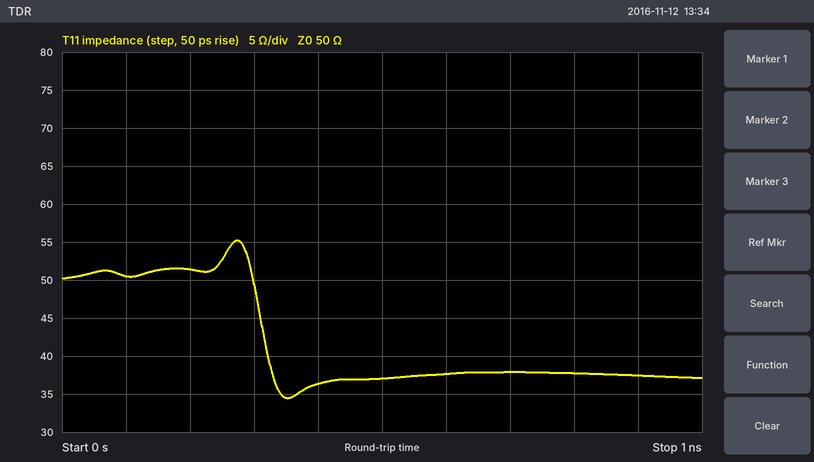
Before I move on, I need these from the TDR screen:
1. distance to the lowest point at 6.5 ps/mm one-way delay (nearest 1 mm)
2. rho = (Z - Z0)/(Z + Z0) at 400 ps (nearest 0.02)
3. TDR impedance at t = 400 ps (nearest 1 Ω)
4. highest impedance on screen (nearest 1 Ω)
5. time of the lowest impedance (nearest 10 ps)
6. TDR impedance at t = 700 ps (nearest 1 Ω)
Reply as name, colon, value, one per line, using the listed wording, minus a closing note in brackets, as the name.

distance to the lowest point at 6.5 ps/mm one-way delay: 27 mm
rho = (Z - Z0)/(Z + Z0) at 400 ps: -0.16
TDR impedance at t = 400 ps: 36 Ω
highest impedance on screen: 55 Ω
time of the lowest impedance: 350 ps
TDR impedance at t = 700 ps: 38 Ω
